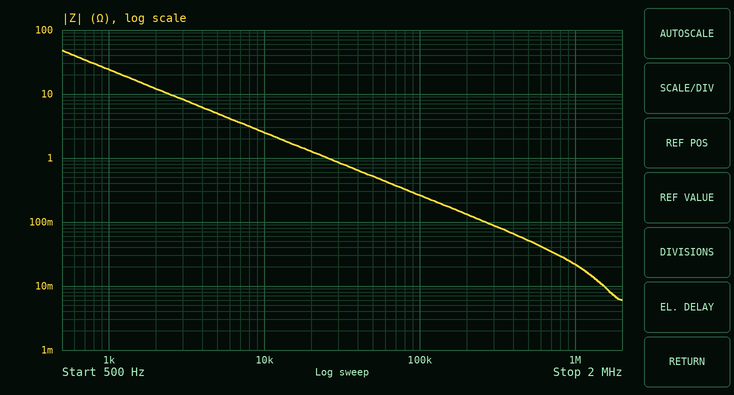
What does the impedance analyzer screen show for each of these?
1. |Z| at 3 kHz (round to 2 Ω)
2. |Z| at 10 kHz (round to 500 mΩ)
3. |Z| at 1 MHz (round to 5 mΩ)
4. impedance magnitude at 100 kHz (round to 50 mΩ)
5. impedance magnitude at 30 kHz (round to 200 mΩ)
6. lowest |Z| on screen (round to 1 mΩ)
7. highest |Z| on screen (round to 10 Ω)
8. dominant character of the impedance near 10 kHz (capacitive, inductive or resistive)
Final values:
8 Ω
2.5 Ω
20 mΩ
250 mΩ
800 mΩ
6 mΩ
50 Ω
capacitive
